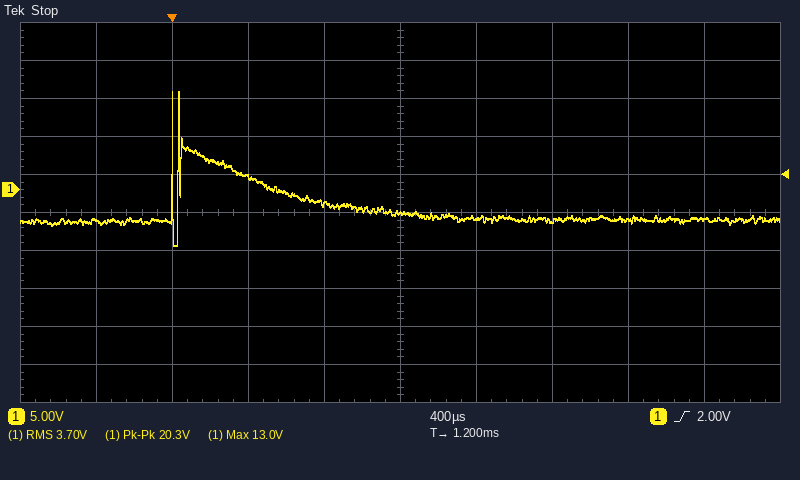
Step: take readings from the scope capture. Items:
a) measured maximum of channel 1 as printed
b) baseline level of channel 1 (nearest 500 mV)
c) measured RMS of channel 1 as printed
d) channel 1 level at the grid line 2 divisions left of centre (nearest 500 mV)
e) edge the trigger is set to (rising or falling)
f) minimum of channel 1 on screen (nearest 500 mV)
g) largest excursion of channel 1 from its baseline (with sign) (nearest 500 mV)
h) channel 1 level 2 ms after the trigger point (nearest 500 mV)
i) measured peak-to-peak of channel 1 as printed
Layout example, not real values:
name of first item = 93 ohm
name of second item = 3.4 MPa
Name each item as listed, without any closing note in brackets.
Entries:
measured maximum of channel 1 as printed = 13.0 V
baseline level of channel 1 = -4.0 V
measured RMS of channel 1 as printed = 3.70 V
channel 1 level at the grid line 2 divisions left of centre = 1.5 V
edge the trigger is set to = rising
minimum of channel 1 on screen = -7.5 V
largest excursion of channel 1 from its baseline (with sign) = +17.0 V
channel 1 level 2 ms after the trigger point = -4.0 V
measured peak-to-peak of channel 1 as printed = 20.3 V
